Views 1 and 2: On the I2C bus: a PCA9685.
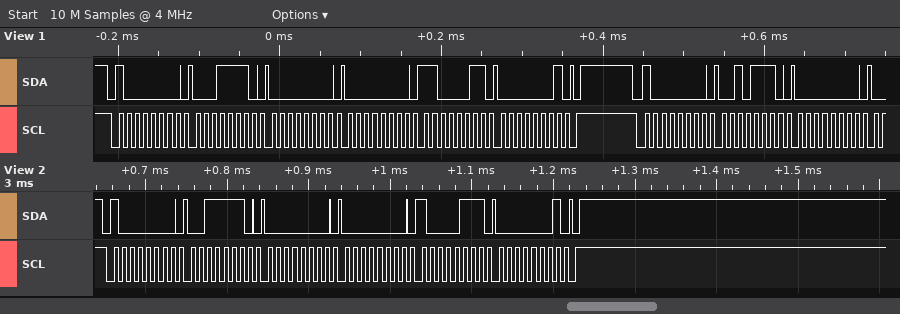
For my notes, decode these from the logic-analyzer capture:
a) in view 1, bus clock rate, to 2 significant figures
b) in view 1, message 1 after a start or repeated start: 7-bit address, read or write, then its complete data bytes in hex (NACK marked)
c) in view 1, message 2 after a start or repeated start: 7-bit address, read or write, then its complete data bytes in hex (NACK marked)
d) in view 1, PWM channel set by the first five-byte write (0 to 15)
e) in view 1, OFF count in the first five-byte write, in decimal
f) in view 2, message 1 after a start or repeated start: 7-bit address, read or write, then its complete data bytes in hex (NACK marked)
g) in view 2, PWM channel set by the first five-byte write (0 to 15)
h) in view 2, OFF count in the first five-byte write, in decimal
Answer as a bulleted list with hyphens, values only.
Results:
- 100 kHz
- 0x40 write: 1E 00 00 C3 01
- 0x40 write: 2E 00
- 6
- 451
- 0x40 write: 3E 00 00 87 01
- 14
- 391
